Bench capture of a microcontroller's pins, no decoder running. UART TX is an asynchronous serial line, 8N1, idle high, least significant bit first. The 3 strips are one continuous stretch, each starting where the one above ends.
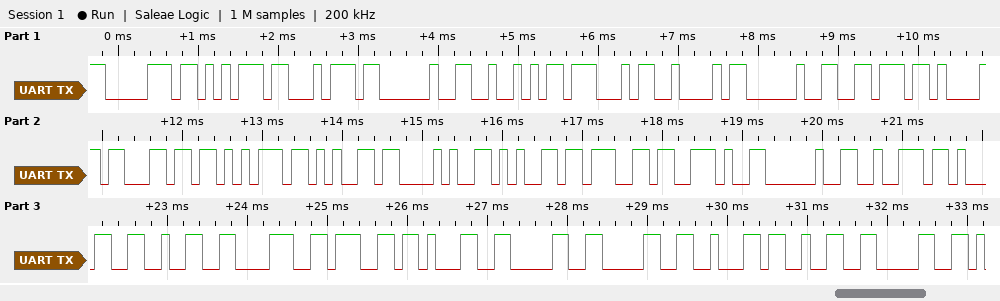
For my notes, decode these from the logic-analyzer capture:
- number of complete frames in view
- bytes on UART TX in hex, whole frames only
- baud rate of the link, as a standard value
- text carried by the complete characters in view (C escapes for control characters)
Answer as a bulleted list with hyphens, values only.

- 29
- 70 75 74 20 52 47 42 20 76 61 6C 75 65 28 65 67 2E 20 72 31 32 38 67 31 30 30 62 32 30
- 9600 baud
- "put RGB value(eg. r128g100b20"
